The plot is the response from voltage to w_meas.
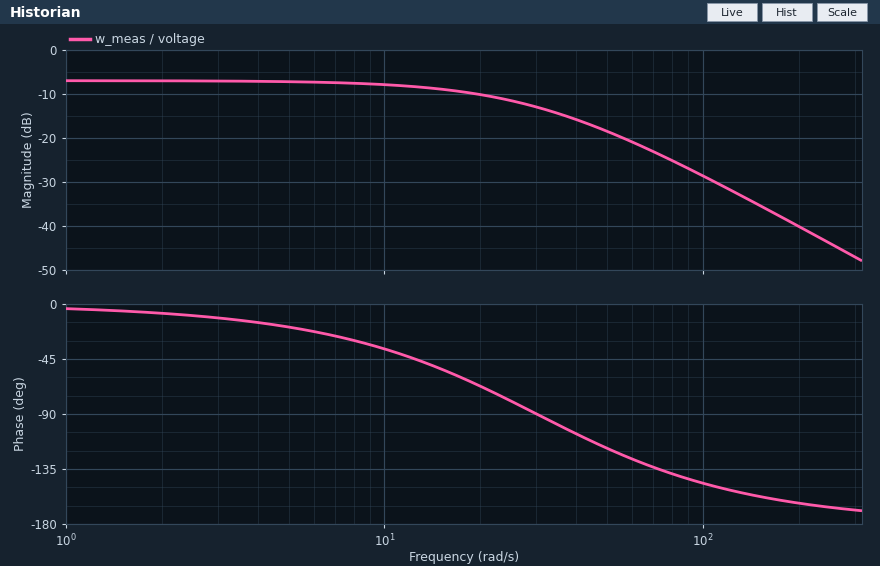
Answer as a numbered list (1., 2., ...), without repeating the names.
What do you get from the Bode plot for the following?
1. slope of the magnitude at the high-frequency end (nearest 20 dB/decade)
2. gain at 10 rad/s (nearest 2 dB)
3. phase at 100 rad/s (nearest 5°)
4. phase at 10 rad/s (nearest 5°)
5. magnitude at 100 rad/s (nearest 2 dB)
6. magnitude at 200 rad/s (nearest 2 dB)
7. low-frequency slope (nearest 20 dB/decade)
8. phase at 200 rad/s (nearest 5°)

1. -40 dB/decade
2. -8 dB
3. -145°
4. -35°
5. -28 dB
6. -40 dB
7. 0 dB/decade
8. -165°
